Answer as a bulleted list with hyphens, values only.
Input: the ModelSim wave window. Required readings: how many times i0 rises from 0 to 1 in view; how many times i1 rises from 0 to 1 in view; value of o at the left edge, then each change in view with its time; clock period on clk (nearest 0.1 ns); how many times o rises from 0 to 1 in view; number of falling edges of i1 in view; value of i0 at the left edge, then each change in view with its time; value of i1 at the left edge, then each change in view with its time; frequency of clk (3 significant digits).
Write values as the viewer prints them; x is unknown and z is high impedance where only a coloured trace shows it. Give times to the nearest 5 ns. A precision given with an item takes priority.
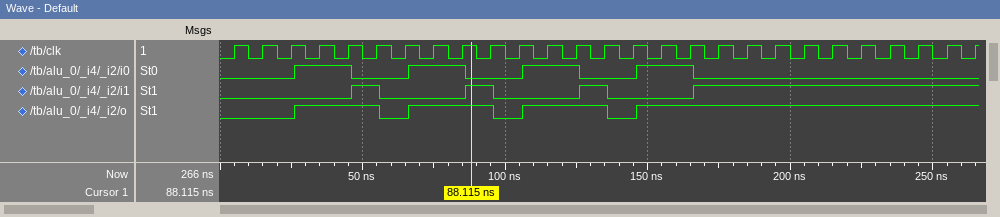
- 4
- 4
- 0, 1 at 25 ns, 0 at 55 ns, 1 at 65 ns, 0 at 95 ns, 1 at 105 ns, 0 at 135 ns, 1 at 145 ns
- 10 ns
- 4
- 3
- 0, 1 at 25 ns, 0 at 45 ns, 1 at 65 ns, 0 at 85 ns, 1 at 105 ns, 0 at 125 ns, 1 at 145 ns, 0 at 165 ns
- 0, 1 at 45 ns, 0 at 55 ns, 1 at 85 ns, 0 at 95 ns, 1 at 125 ns, 0 at 135 ns, 1 at 165 ns
- 100 MHz
